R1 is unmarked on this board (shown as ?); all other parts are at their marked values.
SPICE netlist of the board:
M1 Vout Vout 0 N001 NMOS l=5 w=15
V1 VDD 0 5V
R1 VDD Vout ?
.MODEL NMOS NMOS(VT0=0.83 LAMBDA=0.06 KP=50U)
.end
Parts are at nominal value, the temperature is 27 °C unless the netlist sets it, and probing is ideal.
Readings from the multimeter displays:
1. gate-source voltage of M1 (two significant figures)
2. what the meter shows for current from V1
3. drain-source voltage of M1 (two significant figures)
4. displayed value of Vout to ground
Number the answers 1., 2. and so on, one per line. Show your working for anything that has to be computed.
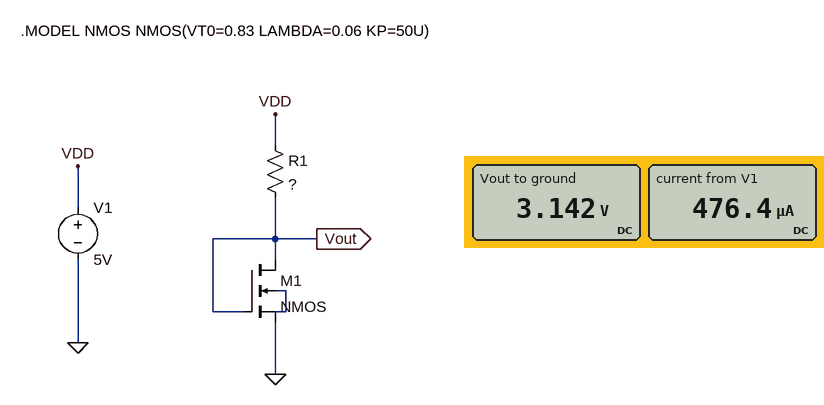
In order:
1. 3.142 V = 3.1 V
2. 476.4 µA
3. 3.142 V = 3.1 V
4. 3.142 V
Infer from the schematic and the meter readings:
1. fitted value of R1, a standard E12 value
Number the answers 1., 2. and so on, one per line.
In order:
1. 3.9 kΩ
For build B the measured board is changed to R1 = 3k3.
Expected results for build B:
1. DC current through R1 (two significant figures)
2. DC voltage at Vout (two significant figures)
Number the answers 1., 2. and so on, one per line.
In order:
1. 530 µA
2. 3.3 V
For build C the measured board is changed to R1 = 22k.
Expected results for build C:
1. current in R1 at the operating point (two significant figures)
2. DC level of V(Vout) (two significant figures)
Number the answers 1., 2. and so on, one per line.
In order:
1. 130 µA
2. 2.1 V
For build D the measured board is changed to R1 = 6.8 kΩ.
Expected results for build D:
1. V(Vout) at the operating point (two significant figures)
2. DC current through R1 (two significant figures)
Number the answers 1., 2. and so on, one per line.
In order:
1. 2.8 V
2. 330 µA
